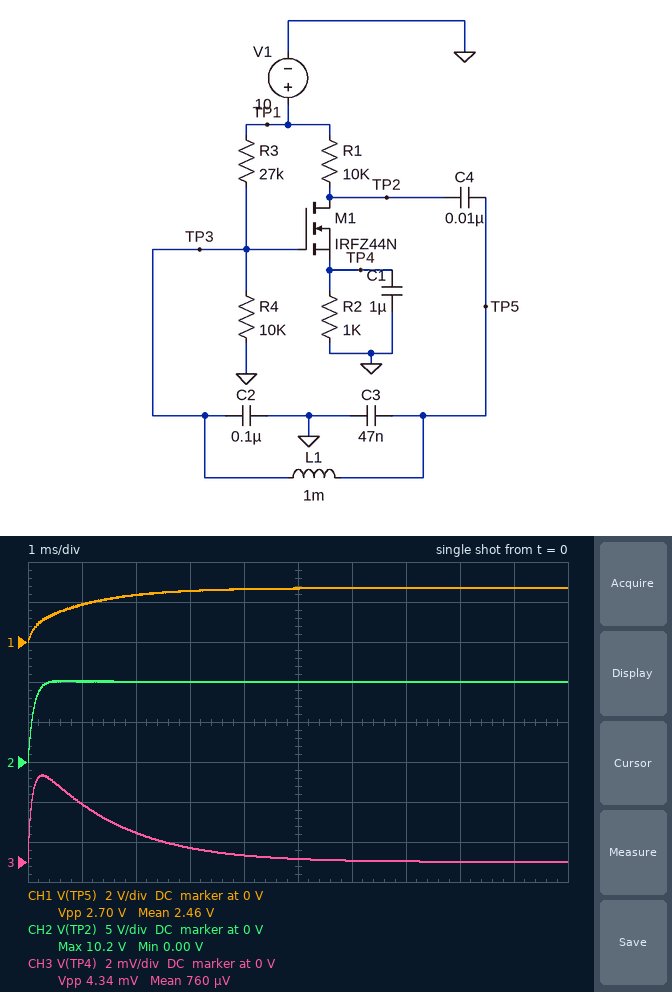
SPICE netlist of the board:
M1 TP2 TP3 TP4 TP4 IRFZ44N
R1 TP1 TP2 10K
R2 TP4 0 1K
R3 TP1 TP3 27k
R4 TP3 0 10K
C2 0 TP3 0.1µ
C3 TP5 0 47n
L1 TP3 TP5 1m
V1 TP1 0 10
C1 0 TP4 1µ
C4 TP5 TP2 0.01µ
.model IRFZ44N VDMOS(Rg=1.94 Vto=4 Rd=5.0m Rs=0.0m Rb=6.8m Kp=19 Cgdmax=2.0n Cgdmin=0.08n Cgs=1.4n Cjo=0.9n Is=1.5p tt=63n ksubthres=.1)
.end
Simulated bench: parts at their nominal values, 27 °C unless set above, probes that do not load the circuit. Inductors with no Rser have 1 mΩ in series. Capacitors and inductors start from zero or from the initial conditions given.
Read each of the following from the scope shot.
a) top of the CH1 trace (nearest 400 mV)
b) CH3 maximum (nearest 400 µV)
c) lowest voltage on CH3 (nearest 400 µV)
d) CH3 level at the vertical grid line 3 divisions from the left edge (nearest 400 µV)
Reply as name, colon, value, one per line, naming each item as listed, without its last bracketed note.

top of the CH1 trace: 2.8 V
CH3 maximum: 4.4 mV
lowest voltage on CH3: 0 V
CH3 level at the vertical grid line 3 divisions from the left edge: 800 µV
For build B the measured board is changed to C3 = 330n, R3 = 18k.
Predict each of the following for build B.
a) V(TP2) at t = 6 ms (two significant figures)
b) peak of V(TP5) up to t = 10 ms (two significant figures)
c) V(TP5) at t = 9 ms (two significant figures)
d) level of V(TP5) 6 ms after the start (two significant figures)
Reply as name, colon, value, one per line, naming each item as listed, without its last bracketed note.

V(TP2) at t = 6 ms: 10 V
peak of V(TP5) up to t = 10 ms: 3.5 V
V(TP5) at t = 9 ms: 3.4 V
level of V(TP5) 6 ms after the start: 3.2 V
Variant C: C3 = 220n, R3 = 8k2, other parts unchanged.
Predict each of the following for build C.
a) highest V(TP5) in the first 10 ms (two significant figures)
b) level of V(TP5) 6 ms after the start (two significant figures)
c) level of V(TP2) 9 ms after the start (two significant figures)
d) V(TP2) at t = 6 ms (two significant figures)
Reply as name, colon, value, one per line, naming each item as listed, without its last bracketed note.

highest V(TP5) in the first 10 ms: 5.5 V
level of V(TP5) 6 ms after the start: 5.4 V
level of V(TP2) 9 ms after the start: 910 mV
V(TP2) at t = 6 ms: 900 mV
